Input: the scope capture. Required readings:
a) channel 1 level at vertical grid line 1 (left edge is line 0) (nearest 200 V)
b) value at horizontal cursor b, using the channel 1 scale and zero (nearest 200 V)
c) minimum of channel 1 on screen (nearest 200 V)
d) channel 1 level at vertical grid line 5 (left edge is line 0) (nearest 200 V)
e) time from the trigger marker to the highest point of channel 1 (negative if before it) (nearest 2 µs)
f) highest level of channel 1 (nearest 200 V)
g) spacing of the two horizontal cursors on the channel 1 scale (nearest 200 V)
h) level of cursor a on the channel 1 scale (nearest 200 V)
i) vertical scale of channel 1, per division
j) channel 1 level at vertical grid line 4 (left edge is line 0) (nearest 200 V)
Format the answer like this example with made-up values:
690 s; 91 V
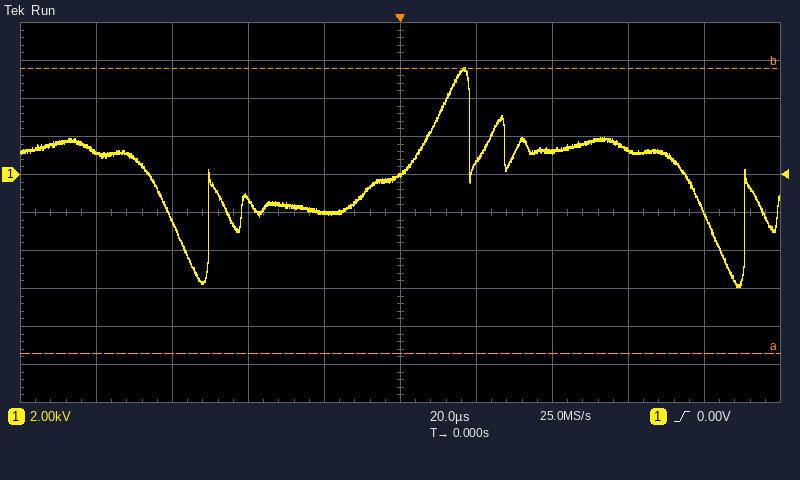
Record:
1.2 kV; 5.6 kV; -5.8 kV; 0.0 kV; +16 µs; 5.6 kV; 15.0 kV; -9.4 kV; 2 kV; -2.0 kV
